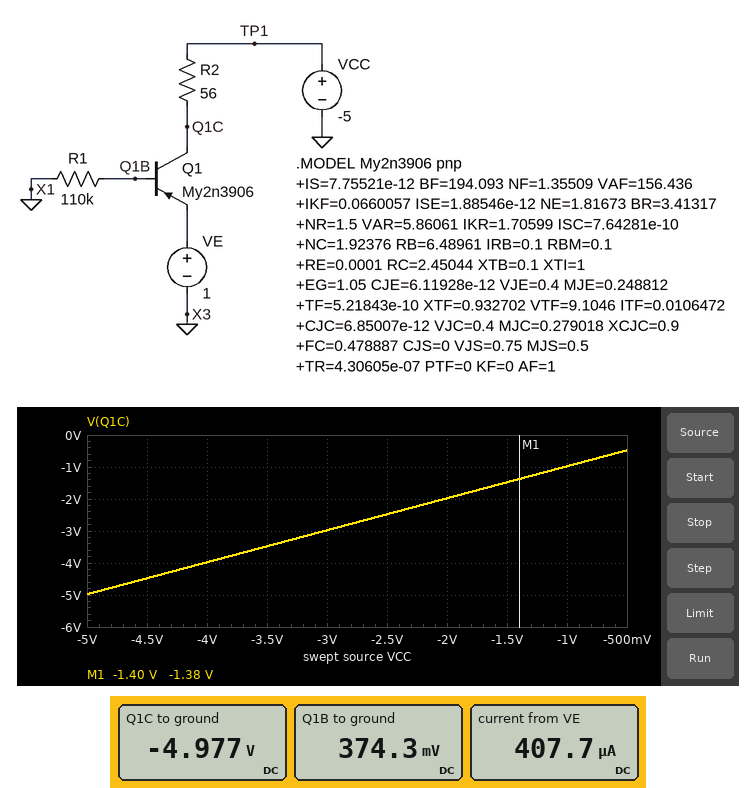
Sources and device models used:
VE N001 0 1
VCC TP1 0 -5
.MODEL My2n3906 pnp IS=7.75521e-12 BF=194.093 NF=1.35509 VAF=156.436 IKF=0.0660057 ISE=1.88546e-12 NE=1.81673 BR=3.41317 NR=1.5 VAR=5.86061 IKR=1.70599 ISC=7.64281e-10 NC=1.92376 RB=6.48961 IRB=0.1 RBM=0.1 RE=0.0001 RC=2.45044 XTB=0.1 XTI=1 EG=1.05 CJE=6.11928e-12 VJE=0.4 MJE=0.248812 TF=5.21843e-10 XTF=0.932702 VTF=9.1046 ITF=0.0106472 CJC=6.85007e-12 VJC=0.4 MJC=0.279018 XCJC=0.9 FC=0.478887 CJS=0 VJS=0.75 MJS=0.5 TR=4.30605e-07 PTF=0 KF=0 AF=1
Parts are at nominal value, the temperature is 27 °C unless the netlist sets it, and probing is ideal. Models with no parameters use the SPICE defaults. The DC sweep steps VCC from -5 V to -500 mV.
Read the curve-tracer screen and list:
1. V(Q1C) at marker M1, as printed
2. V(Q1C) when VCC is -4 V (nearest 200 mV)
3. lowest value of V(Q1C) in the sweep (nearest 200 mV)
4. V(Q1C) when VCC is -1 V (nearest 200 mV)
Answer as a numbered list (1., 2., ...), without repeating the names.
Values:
1. -1.38 V
2. -4.0 V
3. -5.0 V
4. -1.0 V
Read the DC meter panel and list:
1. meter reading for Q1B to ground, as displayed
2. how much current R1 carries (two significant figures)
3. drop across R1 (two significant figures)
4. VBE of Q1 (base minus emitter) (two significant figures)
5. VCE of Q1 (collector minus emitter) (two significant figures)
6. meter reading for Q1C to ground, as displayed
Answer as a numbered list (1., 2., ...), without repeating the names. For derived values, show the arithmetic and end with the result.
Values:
1. 374.3 mV
2. (374.3 mV) / 110 kΩ = 3.4 µA
3. 374.3 mV = 370 mV
4. 374.3 mV - 1 V = -630 mV
5. -4.977 V - 1 V = -6.0 V
6. -4.977 V
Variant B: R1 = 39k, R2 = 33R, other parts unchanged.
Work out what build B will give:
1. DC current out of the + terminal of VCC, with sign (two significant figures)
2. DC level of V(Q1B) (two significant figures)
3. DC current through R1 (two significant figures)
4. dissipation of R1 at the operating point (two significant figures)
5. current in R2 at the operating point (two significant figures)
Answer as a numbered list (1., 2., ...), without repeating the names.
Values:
1. -1.1 mA
2. 340 mV
3. 8.7 µA
4. 2.9 µW
5. 1.1 mA
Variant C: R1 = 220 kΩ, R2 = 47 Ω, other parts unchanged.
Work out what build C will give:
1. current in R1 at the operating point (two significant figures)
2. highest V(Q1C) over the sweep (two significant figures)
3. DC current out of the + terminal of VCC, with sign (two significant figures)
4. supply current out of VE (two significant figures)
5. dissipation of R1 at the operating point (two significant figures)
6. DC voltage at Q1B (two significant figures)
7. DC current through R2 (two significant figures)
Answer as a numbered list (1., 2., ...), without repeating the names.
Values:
1. 1.8 µA
2. -490 mV
3. -200 µA
4. 210 µA
5. 720 nW
6. 400 mV
7. 200 µA
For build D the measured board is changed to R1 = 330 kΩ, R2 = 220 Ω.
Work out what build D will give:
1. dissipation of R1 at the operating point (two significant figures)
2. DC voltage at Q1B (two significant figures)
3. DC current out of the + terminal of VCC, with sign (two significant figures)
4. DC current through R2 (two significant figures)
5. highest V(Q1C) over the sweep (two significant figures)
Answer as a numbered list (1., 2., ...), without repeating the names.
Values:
1. 520 nW
2. 410 mV
3. -140 µA
4. 140 µA
5. -470 mV
